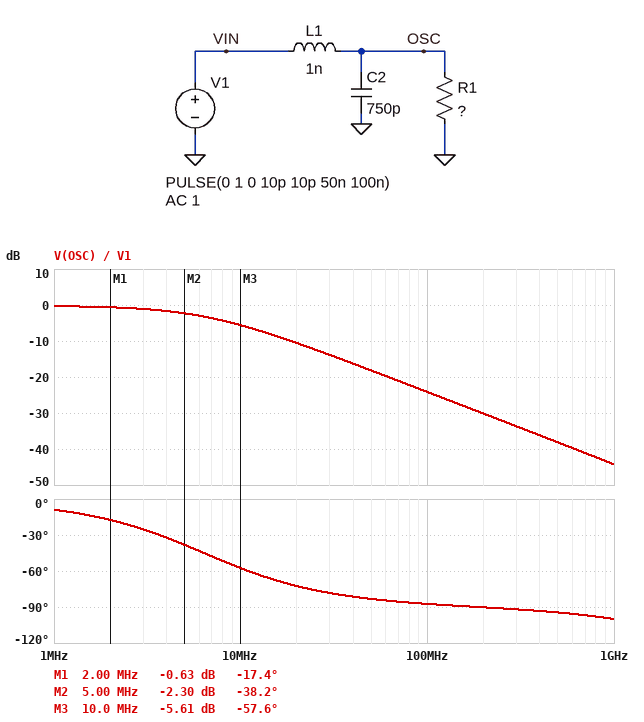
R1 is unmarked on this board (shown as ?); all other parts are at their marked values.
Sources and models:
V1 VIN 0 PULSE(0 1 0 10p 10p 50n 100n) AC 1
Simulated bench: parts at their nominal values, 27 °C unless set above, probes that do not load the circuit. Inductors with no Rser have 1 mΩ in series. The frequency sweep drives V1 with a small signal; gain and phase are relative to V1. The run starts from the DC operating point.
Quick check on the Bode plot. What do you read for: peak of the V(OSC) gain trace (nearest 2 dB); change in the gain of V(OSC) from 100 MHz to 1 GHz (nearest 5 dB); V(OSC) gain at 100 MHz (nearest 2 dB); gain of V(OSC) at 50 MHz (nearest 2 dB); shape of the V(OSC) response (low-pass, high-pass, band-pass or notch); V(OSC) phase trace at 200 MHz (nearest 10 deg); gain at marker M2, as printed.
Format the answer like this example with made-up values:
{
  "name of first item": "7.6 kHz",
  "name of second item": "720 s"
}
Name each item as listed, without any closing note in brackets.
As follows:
{
  "peak of the V(OSC) gain trace": "0 dB",
  "change in the gain of V(OSC) from 100 MHz to 1 GHz": "-20 dB",
  "V(OSC) gain at 100 MHz": "-24 dB",
  "gain of V(OSC) at 50 MHz": "-18 dB",
  "shape of the V(OSC) response": "low-pass",
  "V(OSC) phase trace at 200 MHz": "-90 deg",
  "gain at marker M2, as printed": "-2.30 dB"
}
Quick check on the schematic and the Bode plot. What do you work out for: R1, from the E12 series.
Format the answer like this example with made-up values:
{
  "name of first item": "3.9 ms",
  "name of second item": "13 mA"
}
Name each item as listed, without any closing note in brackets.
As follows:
{
  "R1, from the E12 series": "0.039 Ω"
}
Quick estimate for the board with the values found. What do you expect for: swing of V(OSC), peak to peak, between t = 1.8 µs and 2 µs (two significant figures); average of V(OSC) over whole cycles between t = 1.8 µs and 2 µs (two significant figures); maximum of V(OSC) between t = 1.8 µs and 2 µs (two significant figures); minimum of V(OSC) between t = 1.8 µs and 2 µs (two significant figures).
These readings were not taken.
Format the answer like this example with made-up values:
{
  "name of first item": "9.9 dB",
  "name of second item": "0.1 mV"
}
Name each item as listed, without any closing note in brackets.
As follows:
{
  "swing of V(OSC), peak to peak, between t = 1.8 µs and 2 µs": "740 mV",
  "average of V(OSC) over whole cycles between t = 1.8 µs and 2 µs": "490 mV",
  "maximum of V(OSC) between t = 1.8 µs and 2 µs": "860 mV",
  "minimum of V(OSC) between t = 1.8 µs and 2 µs": "120 mV"
}
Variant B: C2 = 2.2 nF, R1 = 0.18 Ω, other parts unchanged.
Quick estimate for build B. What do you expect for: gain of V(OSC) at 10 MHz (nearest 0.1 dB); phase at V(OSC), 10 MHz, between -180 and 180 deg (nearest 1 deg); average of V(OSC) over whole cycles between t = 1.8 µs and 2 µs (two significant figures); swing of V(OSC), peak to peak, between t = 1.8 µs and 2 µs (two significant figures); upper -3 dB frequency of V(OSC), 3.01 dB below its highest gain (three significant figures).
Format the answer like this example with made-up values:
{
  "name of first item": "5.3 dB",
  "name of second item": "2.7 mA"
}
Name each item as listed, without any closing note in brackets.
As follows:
{
  "gain of V(OSC) at 10 MHz": "-0.5 dB",
  "phase at V(OSC), 10 MHz, between -180 and 180 deg": "-19 deg",
  "average of V(OSC) over whole cycles between t = 1.8 µs and 2 µs": "500 mV",
  "swing of V(OSC), peak to peak, between t = 1.8 µs and 2 µs": "990 mV",
  "upper -3 dB frequency of V(OSC), 3.01 dB below its highest gain": "31.0 MHz"
}
